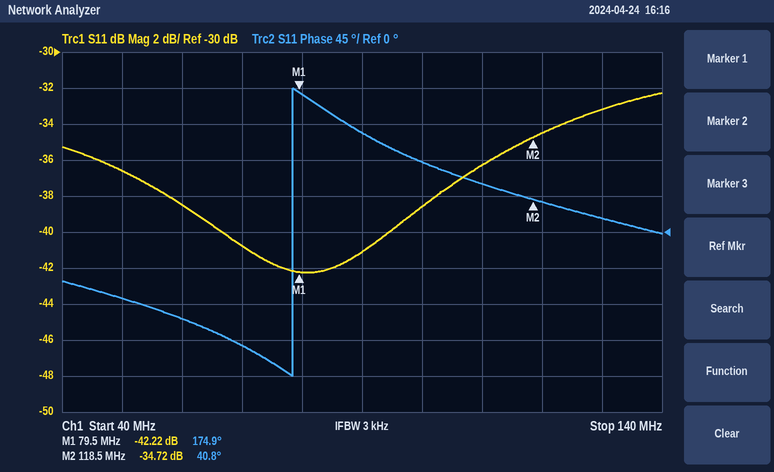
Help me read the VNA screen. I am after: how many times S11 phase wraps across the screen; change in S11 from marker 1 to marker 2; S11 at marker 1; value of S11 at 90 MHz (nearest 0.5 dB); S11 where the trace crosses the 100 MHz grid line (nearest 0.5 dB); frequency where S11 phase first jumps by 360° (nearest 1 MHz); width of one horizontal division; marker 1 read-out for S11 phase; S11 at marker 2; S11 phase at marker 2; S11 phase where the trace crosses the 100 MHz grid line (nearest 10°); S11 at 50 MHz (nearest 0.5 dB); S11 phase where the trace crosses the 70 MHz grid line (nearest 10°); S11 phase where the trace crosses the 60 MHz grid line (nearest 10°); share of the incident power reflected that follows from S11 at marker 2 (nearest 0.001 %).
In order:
1
7.50 dB
-42.22 dB
-41.0 dB
-38.5 dB
78 MHz
10 MHz
174.9°
-34.72 dB
40.8°
90°
-36.5 dB
-140°
-110°
0.034 %
